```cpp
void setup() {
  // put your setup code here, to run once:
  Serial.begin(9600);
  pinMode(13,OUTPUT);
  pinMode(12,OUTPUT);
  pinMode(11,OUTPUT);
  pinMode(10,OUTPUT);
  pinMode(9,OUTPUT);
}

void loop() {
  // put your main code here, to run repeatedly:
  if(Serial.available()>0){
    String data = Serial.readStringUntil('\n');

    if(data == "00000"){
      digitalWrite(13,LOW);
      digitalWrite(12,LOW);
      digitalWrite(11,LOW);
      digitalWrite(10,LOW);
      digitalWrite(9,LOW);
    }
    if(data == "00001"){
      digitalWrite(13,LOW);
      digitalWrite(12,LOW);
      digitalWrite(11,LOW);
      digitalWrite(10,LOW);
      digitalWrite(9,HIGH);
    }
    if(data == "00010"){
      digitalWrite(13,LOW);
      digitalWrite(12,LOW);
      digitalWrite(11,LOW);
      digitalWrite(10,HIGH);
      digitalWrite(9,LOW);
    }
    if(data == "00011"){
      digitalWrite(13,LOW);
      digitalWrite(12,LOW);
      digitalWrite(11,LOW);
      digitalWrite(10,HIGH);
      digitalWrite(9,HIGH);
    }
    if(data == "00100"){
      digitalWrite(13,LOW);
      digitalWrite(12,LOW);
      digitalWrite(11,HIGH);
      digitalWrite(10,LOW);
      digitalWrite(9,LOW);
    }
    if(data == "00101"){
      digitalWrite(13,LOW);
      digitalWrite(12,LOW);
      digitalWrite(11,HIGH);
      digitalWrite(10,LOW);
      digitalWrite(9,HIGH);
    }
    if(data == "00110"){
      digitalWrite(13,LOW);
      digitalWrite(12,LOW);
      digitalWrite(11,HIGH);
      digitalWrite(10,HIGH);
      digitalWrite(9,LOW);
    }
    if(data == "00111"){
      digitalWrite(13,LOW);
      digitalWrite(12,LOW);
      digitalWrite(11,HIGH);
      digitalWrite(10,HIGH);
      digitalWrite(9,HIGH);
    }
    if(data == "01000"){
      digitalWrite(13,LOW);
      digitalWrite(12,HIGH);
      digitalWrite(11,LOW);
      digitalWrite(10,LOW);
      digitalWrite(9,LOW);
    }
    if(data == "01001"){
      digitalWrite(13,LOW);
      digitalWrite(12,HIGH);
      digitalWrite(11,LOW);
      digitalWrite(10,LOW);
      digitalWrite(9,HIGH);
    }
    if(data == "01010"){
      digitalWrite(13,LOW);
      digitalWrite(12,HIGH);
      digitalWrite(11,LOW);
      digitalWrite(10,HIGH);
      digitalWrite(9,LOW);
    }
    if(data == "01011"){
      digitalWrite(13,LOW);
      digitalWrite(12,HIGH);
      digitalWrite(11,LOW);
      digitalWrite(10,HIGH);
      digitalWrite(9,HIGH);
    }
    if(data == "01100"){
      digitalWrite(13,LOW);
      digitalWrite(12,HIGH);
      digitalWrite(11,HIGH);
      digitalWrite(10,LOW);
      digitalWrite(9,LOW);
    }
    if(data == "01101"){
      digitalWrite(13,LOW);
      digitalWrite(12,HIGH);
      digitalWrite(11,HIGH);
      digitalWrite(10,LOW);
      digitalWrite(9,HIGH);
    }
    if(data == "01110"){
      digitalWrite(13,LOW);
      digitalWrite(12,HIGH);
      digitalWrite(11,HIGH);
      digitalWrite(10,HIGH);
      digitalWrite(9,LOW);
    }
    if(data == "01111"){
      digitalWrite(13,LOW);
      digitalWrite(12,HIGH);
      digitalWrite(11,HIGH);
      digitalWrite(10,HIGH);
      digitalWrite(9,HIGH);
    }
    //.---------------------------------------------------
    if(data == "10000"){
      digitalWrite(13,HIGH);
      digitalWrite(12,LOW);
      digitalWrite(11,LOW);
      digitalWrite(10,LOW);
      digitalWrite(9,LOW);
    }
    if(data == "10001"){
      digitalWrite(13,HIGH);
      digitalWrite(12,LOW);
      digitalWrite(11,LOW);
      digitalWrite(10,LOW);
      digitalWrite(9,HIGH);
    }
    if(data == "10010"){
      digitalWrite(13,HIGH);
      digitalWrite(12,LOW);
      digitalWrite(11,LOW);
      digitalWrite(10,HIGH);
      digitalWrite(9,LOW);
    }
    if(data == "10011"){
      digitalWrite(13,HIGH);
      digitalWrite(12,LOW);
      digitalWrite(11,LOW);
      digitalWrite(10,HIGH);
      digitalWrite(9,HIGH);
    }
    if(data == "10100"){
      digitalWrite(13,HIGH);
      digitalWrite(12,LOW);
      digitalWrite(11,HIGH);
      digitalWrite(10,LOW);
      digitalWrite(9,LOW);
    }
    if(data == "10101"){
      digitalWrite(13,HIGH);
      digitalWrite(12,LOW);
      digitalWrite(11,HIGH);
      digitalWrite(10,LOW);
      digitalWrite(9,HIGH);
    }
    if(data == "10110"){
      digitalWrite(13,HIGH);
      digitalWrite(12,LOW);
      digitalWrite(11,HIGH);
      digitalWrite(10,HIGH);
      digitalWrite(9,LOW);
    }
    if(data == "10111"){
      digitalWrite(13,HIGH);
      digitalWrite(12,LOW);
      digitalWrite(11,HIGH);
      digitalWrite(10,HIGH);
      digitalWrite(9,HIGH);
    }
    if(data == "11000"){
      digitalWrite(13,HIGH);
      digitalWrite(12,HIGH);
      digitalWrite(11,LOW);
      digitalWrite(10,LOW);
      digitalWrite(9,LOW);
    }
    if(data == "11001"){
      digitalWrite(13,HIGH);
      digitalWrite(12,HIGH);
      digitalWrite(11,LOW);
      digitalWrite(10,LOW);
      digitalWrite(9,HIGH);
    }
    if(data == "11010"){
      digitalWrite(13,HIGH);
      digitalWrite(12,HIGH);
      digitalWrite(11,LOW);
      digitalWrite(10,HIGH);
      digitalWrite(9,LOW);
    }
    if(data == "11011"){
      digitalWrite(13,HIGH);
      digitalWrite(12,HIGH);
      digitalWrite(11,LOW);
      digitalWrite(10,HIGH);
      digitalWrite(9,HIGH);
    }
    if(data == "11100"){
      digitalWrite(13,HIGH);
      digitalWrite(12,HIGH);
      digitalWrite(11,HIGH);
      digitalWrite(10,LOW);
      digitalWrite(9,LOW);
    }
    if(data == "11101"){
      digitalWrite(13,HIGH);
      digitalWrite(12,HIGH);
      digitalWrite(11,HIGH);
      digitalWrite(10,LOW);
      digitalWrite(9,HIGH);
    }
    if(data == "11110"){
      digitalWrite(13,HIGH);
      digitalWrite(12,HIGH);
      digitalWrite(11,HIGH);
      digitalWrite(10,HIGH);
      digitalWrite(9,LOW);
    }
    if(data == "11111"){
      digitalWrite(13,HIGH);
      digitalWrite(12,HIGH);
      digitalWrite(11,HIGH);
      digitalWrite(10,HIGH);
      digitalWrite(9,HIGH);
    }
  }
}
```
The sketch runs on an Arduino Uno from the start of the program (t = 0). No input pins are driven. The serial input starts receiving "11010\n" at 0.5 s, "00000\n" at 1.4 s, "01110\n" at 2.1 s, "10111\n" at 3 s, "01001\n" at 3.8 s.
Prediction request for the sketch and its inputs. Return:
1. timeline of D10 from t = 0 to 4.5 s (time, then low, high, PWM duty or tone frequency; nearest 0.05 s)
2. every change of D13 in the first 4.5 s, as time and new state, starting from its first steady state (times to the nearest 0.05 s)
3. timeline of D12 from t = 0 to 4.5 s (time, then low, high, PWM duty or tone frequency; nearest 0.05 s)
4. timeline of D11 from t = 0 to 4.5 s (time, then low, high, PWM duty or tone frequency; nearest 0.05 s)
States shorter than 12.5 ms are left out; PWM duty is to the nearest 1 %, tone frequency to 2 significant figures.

0 s low; 0.5 s high; 1.4 s low; 2.1 s high; 3.8 s low
0 s low; 0.5 s high; 1.4 s low; 3 s high; 3.8 s low
0 s low; 0.5 s high; 1.4 s low; 2.1 s high; 3 s low; 3.8 s high
0 s low; 2.1 s high; 3.8 s low
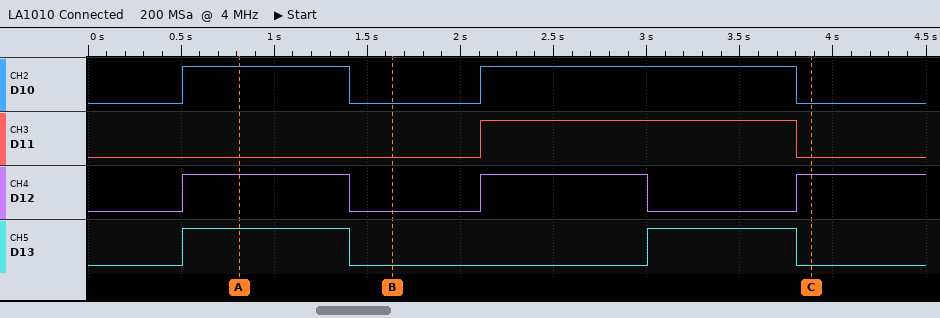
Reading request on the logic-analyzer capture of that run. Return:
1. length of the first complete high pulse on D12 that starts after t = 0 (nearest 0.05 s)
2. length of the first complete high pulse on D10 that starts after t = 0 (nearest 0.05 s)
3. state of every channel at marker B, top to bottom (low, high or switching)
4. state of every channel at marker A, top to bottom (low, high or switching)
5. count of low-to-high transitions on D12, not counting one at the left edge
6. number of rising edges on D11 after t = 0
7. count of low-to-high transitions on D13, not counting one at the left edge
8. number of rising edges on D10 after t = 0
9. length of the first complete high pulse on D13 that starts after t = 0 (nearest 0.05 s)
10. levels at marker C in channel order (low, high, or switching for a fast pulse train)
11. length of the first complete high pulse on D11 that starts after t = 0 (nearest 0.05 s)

0.90 s
0.90 s
D10 low, D11 low, D12 low, D13 low
D10 high, D11 low, D12 high, D13 high
3
1
2
2
0.90 s
D10 low, D11 low, D12 high, D13 low
1.70 s
